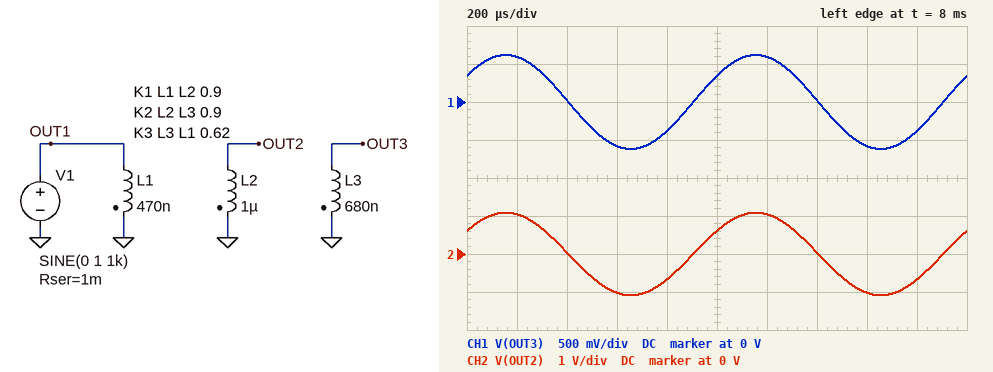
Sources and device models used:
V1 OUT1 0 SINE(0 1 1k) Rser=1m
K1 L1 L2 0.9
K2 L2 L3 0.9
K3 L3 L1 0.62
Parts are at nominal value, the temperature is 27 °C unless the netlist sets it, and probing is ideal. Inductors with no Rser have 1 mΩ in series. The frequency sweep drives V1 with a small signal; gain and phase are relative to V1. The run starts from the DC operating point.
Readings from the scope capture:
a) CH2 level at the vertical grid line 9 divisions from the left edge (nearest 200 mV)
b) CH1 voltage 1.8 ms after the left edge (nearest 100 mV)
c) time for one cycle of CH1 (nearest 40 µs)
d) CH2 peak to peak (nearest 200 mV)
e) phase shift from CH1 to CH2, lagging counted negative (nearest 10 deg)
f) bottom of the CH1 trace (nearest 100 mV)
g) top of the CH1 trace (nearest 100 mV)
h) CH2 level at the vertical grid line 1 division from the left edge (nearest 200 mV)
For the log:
-600 mV
-400 mV
1.00 ms
2.2 V
0 deg
-600 mV
600 mV
1.0 V
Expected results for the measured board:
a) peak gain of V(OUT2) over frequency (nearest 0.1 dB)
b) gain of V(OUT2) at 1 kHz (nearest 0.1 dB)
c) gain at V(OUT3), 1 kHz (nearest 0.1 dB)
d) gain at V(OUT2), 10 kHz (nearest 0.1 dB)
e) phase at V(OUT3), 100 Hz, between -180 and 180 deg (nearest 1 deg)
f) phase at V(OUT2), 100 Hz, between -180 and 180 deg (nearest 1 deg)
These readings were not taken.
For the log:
2.4 dB
0.7 dB
-4.2 dB
2.3 dB
82 deg
82 deg
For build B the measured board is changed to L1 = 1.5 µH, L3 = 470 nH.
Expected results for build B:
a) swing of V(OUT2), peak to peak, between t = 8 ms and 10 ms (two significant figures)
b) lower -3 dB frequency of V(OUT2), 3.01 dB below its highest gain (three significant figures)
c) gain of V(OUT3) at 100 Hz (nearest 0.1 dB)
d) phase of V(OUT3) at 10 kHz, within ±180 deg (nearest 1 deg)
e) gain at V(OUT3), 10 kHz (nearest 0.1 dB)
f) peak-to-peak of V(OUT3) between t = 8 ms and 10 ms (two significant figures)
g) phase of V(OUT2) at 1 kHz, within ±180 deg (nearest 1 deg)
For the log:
1.4 V
212 Hz
-16.6 dB
1 deg
-9.2 dB
680 mV
12 deg
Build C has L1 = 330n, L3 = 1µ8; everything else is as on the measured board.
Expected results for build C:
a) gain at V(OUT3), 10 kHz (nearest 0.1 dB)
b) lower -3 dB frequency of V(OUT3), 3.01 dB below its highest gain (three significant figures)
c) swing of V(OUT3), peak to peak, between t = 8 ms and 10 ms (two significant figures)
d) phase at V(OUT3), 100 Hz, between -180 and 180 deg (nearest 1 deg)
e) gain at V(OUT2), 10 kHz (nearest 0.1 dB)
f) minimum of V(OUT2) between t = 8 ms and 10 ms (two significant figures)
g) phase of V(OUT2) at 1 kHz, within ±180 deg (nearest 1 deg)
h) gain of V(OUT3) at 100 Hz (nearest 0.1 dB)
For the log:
3.2 dB
965 Hz
2.1 V
84 deg
3.9 dB
-1.1 V
44 deg
-16.5 dB
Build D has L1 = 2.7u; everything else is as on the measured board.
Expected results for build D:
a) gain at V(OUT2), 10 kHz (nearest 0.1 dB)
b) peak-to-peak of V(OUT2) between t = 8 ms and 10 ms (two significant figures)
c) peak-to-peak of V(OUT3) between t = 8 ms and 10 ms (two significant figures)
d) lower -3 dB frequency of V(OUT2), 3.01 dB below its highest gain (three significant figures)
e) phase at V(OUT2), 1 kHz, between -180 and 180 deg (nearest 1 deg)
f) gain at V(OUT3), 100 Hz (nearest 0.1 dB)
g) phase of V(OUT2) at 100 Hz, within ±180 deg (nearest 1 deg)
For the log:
-5.2 dB
1.1 V
620 mV
118 Hz
7 deg
-13.9 dB
50 deg
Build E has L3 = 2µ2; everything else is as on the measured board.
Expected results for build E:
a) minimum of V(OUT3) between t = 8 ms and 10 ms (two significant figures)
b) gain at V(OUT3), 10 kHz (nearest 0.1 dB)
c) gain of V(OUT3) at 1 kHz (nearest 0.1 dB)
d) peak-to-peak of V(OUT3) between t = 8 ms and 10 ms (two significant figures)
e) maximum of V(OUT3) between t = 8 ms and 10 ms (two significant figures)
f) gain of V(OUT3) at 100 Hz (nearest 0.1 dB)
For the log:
-1.1 V
2.5 dB
0.9 dB
2.2 V
1.1 V
-14.2 dB
